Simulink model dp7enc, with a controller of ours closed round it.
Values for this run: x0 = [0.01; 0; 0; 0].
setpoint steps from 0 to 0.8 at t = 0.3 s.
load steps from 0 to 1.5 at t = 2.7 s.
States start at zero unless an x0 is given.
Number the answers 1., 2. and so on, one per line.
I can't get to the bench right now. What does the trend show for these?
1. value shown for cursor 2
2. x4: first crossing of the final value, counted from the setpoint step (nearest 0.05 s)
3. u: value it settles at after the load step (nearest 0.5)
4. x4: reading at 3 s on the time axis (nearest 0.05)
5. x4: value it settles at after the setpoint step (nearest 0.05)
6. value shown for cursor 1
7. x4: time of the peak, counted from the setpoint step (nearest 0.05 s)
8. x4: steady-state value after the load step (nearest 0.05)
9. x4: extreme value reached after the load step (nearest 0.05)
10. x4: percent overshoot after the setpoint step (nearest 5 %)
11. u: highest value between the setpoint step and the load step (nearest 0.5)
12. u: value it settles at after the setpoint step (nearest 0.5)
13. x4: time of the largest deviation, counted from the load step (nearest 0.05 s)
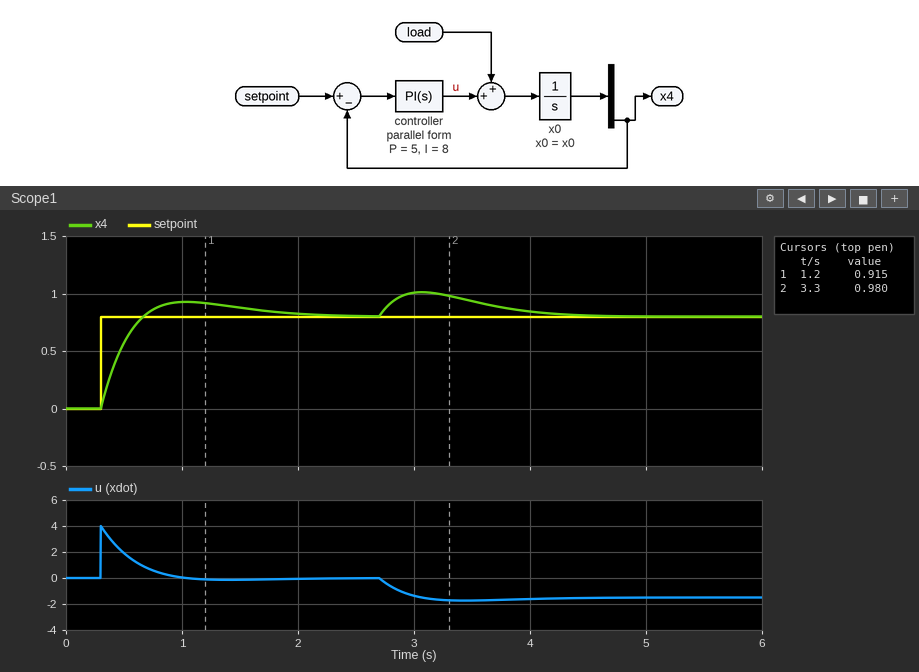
1. 0.980
2. 0.35 s
3. -1.5
4. 1.00
5. 0.80
6. 0.915
7. 0.75 s
8. 0.80
9. 1.00
10. 15 %
11. 4.0
12. 0.0
13. 0.35 s
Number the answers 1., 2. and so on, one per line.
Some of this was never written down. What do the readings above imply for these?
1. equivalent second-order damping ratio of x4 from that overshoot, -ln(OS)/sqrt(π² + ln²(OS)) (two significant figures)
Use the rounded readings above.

1. 0.52
